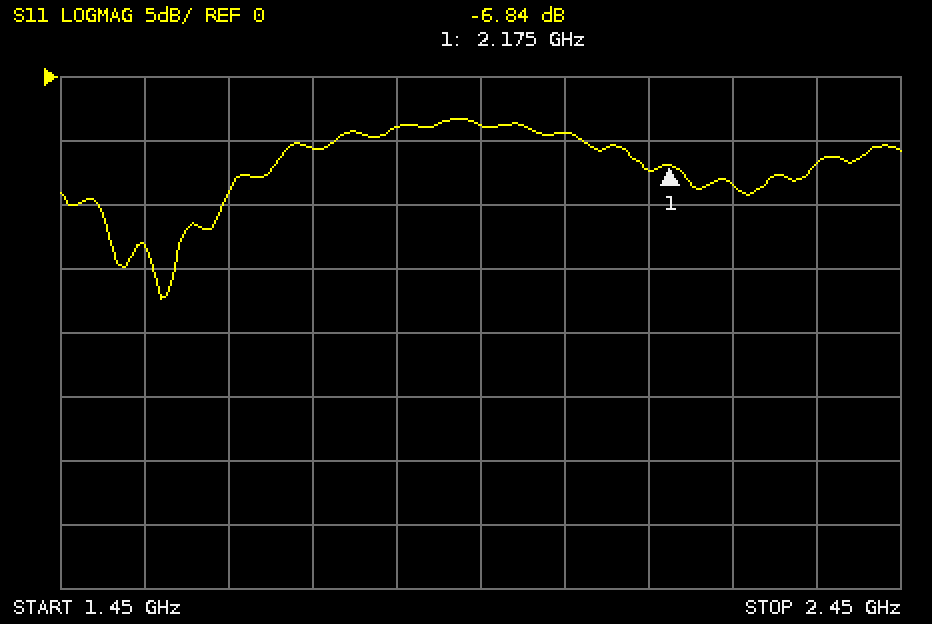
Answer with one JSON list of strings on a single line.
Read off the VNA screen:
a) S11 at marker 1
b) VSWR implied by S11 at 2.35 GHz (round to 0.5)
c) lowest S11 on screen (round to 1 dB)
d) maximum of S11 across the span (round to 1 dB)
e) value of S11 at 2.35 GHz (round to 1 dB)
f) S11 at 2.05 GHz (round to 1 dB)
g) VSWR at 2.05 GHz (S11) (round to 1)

["-6.84 dB", "2.5", "-17 dB", "-3 dB", "-7 dB", "-4 dB", "4"]
